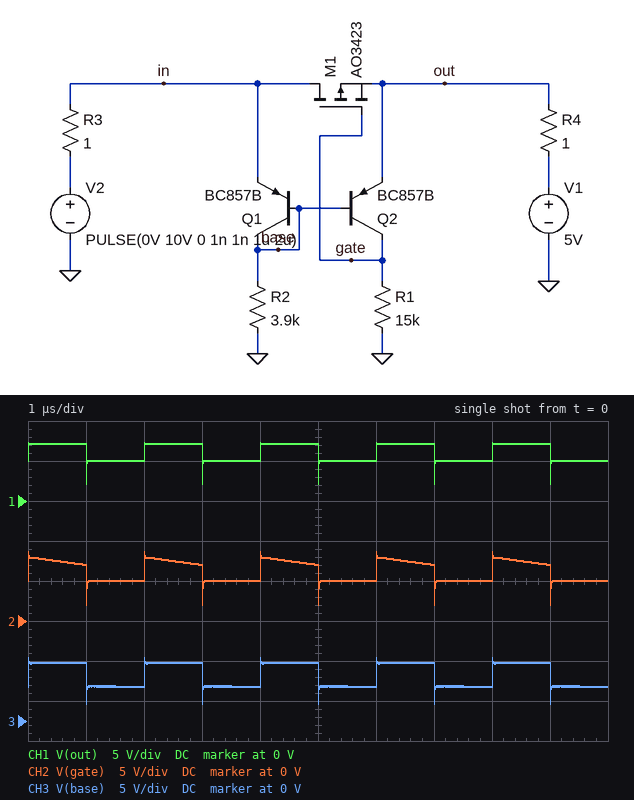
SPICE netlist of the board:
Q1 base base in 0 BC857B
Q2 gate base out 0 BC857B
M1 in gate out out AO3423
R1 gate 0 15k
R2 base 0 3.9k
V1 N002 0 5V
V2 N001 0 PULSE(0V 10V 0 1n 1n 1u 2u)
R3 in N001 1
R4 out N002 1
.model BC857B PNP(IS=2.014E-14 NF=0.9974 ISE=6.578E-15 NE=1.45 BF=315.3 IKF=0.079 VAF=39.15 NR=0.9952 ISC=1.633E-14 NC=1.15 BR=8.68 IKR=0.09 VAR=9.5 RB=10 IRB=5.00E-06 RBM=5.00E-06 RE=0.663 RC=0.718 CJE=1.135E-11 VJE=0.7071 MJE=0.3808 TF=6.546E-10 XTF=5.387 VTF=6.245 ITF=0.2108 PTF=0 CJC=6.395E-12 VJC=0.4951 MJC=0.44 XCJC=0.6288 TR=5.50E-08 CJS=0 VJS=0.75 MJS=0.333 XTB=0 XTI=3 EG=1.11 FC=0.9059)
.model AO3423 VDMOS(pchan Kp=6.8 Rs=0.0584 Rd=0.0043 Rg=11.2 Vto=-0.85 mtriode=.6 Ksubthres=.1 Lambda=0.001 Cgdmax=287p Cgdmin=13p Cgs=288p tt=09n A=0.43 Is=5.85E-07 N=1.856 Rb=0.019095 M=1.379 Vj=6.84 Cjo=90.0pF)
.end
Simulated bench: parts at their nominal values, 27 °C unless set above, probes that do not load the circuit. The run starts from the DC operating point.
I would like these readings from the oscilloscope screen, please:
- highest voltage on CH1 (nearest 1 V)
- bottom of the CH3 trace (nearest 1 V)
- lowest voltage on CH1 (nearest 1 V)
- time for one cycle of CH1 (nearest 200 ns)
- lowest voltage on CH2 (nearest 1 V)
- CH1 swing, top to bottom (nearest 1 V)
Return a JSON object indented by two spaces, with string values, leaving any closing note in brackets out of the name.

{
  "highest voltage on CH1": "7 V",
  "bottom of the CH3 trace": "2 V",
  "lowest voltage on CH1": "2 V",
  "time for one cycle of CH1": "2.0 µs",
  "lowest voltage on CH2": "2 V",
  "CH1 swing, top to bottom": "5 V"
}
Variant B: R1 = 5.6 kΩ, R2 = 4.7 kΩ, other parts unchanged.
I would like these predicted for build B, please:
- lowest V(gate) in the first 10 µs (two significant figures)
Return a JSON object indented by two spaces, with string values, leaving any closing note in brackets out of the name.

{
  "lowest V(gate) in the first 10 µs": "780 mV"
}
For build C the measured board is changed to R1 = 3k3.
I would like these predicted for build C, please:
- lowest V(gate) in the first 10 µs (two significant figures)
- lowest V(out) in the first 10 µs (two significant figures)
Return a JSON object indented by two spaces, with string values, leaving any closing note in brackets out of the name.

{
  "lowest V(gate) in the first 10 µs": "-320 mV",
  "lowest V(out) in the first 10 µs": "2.7 V"
}
